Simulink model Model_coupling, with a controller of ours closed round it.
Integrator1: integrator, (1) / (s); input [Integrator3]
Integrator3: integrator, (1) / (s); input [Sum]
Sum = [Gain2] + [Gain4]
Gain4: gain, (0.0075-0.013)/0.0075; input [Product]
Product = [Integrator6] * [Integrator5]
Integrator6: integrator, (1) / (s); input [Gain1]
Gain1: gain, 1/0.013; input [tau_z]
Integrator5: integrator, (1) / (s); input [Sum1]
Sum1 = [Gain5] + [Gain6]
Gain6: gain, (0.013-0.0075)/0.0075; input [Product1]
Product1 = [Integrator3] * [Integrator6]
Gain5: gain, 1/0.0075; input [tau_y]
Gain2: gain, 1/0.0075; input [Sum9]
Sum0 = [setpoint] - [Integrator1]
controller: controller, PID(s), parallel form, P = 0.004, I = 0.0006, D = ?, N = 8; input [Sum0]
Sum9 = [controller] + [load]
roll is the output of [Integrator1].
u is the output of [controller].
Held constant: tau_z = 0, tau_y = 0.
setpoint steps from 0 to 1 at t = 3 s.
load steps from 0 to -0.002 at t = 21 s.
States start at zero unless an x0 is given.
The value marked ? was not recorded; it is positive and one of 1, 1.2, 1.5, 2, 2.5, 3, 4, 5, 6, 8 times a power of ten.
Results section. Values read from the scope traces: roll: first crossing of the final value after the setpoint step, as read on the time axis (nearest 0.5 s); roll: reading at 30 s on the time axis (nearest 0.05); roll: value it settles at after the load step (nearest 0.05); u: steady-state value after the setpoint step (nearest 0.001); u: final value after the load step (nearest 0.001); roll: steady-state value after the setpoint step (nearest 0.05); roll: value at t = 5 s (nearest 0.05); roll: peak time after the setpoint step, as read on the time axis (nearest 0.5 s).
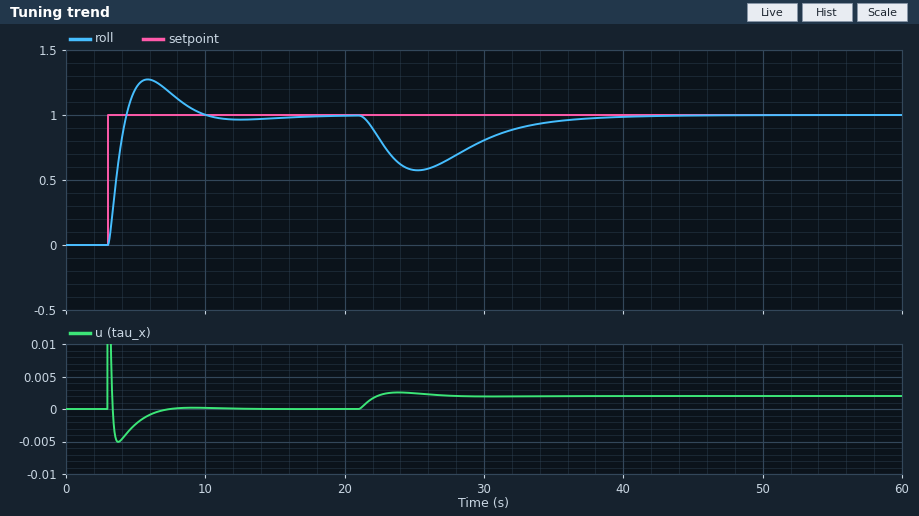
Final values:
4.5 s
0.80
1.00
0.000
0.002
1.00
1.20
6.0 s
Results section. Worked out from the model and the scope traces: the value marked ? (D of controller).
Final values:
0.008
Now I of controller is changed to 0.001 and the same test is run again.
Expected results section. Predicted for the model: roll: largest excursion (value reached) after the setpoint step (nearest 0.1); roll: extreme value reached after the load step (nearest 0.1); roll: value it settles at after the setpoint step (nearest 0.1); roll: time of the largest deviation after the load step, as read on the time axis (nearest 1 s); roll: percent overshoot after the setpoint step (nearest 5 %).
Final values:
1.3
0.6
1.0
25 s
30 %
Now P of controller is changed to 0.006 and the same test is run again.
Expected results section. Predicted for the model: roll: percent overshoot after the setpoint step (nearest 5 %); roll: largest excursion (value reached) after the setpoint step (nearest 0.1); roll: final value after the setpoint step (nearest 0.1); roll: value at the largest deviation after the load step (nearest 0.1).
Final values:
30 %
1.3
1.0
0.7
